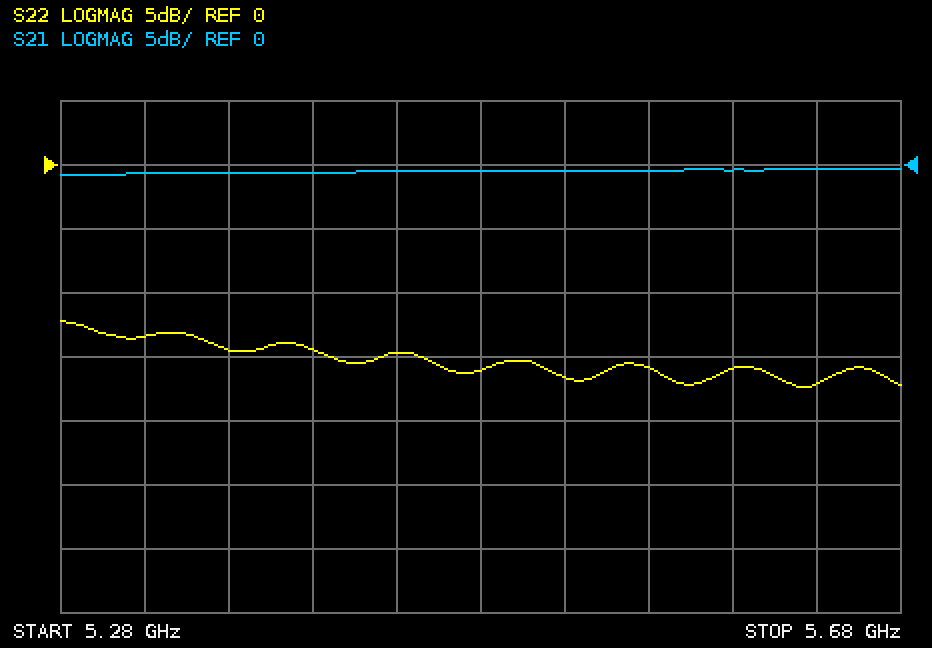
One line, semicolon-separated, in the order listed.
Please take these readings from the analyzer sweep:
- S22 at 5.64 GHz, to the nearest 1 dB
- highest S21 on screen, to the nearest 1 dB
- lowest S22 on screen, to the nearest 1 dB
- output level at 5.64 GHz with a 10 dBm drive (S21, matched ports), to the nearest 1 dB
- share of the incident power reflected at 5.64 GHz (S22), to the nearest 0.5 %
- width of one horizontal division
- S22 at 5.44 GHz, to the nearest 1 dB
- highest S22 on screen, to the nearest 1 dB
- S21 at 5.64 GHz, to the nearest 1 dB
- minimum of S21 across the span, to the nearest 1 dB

-17 dB; 0 dB; -17 dB; 10 dBm; 2.0 %; 40 MHz; -15 dB; -12 dB; 0 dB; -1 dB
